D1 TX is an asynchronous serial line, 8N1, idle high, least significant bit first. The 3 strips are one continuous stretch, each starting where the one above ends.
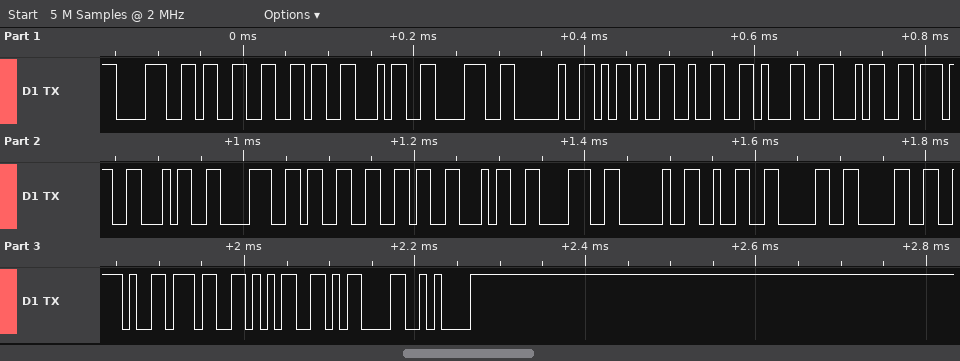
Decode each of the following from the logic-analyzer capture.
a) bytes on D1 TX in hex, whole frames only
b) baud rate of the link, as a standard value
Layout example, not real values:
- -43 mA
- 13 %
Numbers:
- 38 33 36 34 38 20 2D 32 31 34 37 34 38 33 36 34 38 20 32 30 30 2E 37 35 0D 0A
- 115200 baud
